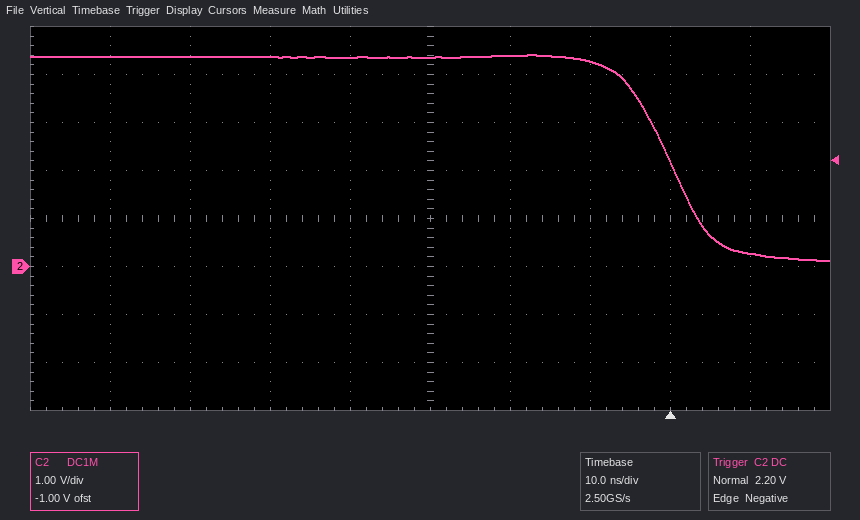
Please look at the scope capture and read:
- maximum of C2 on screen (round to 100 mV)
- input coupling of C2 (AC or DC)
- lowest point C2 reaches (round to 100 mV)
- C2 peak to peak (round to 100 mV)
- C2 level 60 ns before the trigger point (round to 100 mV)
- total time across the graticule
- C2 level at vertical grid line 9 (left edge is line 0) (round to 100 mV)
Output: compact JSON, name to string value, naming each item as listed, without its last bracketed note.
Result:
{"maximum of C2 on screen": "4.4 V", "input coupling of C2": "DC", "lowest point C2 reaches": "100 mV", "C2 peak to peak": "4.3 V", "C2 level 60 ns before the trigger point": "4.4 V", "total time across the graticule": "100 ns", "C2 level at vertical grid line 9 (left edge is line 0)": "300 mV"}
